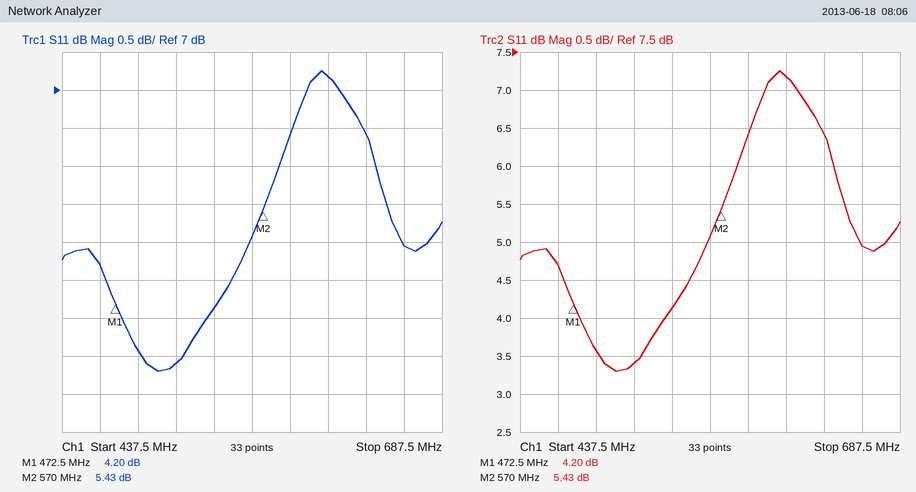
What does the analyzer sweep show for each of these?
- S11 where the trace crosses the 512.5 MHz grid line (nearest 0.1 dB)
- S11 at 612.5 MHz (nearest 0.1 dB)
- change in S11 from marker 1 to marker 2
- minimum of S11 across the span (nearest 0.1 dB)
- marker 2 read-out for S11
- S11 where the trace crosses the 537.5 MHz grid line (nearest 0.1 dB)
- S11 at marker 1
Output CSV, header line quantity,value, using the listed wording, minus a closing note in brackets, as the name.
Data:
quantity,value
S11 where the trace crosses the 512.5 MHz grid line,3.4 dB
S11 at 612.5 MHz,7.2 dB
change in S11 from marker 1 to marker 2,1.23 dB
minimum of S11 across the span,3.3 dB
marker 2 read-out for S11,5.43 dB
S11 where the trace crosses the 537.5 MHz grid line,4.1 dB
S11 at marker 1,4.20 dB
